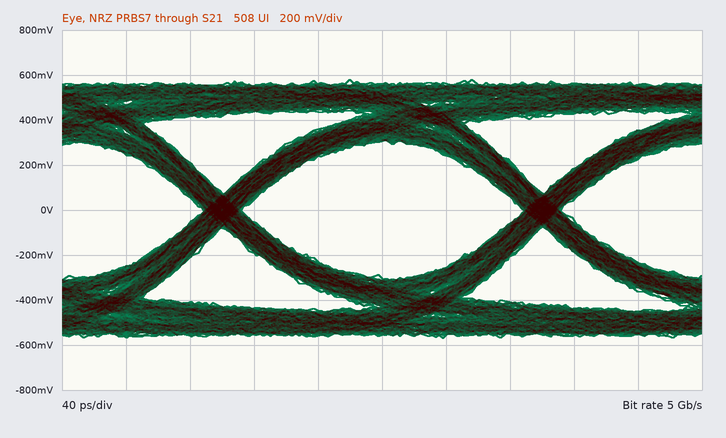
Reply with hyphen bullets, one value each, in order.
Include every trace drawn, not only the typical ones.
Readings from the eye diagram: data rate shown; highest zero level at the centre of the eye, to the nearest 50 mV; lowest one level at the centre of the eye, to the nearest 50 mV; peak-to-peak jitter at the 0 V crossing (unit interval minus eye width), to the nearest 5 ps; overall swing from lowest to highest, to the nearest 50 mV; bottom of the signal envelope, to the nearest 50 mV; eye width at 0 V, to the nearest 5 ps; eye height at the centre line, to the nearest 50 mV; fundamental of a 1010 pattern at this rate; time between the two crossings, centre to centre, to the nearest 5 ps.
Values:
- 5 Gb/s
- -300 mV
- 300 mV
- 25 ps
- 1.15 V
- -550 mV
- 175 ps
- 600 mV
- 2.5 GHz
- 200 ps
